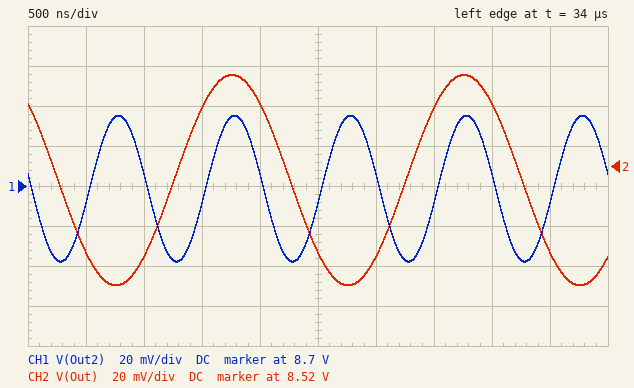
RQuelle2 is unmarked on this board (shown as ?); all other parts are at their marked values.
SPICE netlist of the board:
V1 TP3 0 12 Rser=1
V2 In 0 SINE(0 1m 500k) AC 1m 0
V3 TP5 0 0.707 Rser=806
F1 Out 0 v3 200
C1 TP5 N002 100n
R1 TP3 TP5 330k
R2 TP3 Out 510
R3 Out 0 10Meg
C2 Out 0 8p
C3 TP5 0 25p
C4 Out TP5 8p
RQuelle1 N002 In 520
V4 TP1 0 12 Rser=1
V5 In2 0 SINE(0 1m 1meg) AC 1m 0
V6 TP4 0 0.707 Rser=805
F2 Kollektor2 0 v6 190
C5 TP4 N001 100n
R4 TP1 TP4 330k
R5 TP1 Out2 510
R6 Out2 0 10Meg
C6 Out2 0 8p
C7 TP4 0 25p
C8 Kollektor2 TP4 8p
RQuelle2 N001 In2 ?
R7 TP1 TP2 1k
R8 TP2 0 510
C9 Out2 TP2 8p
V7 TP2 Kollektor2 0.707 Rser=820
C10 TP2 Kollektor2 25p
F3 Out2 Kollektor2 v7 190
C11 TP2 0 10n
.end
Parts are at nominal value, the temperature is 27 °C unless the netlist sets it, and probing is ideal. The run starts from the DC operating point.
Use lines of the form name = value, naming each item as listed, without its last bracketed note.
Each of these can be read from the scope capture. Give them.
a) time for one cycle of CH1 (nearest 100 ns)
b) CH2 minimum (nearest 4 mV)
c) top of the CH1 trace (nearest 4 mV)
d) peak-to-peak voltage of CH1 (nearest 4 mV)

time for one cycle of CH1 = 1.0 µs
CH2 minimum = 8.460 V
top of the CH1 trace = 8.736 V
peak-to-peak voltage of CH1 = 72 mV
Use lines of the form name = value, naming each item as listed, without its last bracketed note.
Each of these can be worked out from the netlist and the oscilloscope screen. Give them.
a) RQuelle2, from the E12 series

RQuelle2, from the E12 series = 1.8 kΩ
